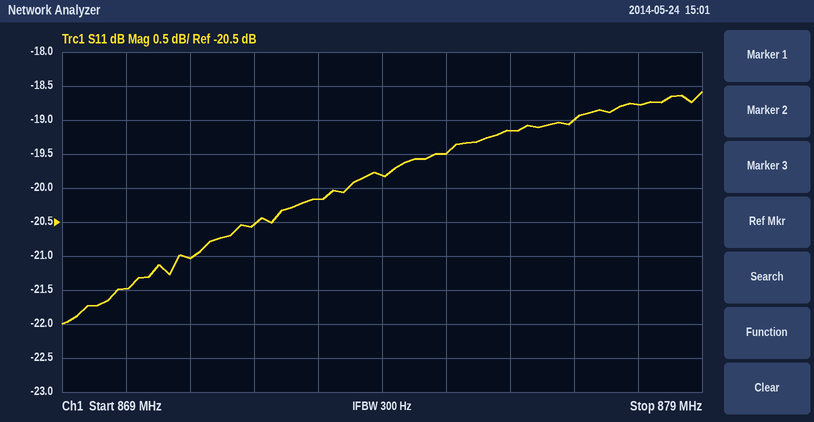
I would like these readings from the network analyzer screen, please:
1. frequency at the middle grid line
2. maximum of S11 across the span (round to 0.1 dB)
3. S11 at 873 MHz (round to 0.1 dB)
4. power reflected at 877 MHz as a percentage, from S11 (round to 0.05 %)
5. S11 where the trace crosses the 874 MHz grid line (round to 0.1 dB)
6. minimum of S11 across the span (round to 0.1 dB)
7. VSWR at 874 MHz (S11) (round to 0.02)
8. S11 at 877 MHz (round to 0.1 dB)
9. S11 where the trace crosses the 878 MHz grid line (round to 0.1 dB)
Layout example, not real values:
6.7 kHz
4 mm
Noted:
874 MHz
-18.6 dB
-20.2 dB
1.25 %
-19.8 dB
-22.0 dB
1.22
-19.0 dB
-18.8 dB
